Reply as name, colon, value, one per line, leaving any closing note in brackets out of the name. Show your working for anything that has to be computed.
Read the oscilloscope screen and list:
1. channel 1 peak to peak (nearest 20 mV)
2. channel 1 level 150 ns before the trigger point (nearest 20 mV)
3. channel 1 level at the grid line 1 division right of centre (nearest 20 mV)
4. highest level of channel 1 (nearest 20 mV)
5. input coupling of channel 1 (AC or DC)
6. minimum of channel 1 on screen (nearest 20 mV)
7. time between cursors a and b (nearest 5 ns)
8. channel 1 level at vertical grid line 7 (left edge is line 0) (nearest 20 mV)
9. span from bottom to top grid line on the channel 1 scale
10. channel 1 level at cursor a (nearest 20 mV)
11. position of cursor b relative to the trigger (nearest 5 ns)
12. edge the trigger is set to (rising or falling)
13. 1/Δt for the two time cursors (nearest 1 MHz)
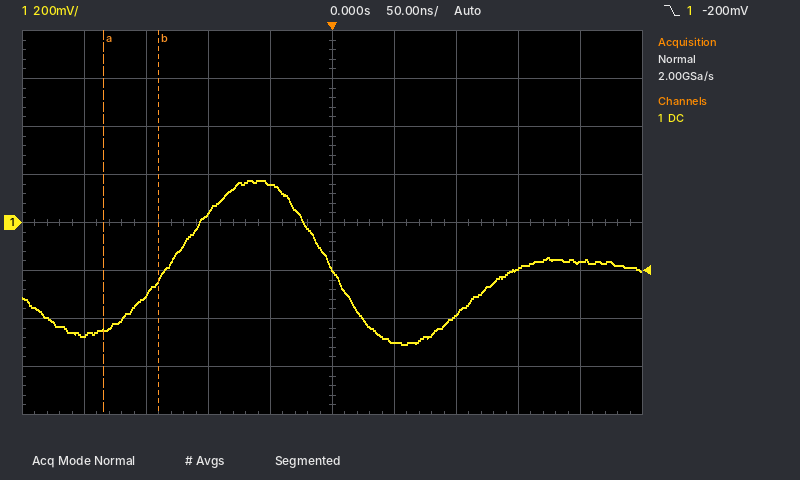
channel 1 peak to peak: 180 mV − (-500 mV) = 680 mV
channel 1 level 150 ns before the trigger point: -300 mV
channel 1 level at the grid line 1 division right of centre: -500 mV
highest level of channel 1: 180 mV
input coupling of channel 1: DC
minimum of channel 1 on screen: -500 mV
time between cursors a and b: 45 ns
channel 1 level at vertical grid line 7 (left edge is line 0): -380 mV
span from bottom to top grid line on the channel 1 scale: 1.6 V
channel 1 level at cursor a: -440 mV
position of cursor b relative to the trigger: -140 ns
edge the trigger is set to: falling
1/Δt for the two time cursors: 1 / 45 ns ≈ 22 MHz
